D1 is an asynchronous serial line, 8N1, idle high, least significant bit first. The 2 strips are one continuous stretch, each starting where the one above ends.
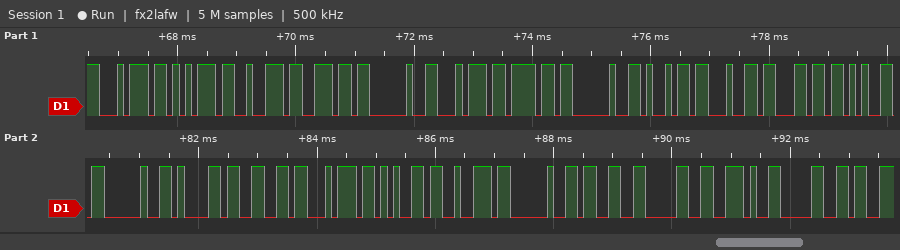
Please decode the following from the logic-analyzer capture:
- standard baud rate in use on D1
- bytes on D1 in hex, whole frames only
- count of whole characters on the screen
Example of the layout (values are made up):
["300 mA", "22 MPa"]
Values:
["9600 baud", "74 75 72 6E 20 74 6F 20 69 64 6C 65 20 61 66 74 65 72 20 33 30 2E 30", "23"]
